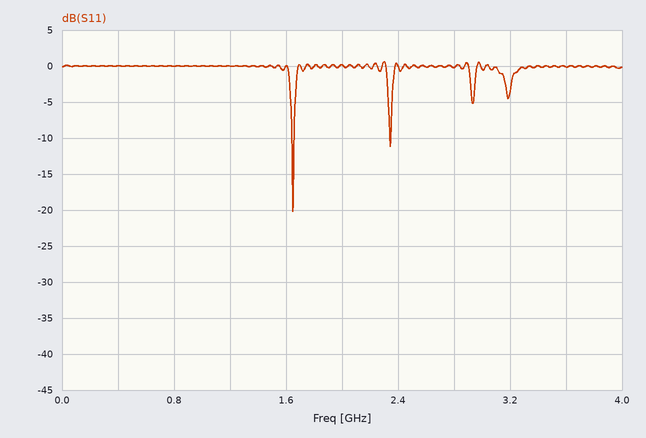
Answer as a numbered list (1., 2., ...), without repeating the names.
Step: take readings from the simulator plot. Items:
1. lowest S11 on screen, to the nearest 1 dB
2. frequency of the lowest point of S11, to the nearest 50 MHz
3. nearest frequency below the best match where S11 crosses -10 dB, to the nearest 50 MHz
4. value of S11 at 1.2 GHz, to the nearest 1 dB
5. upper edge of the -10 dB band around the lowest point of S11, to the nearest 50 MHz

1. -20 dB
2. 1.65 GHz
3. 1.65 GHz
4. 0 dB
5. 1.65 GHz
